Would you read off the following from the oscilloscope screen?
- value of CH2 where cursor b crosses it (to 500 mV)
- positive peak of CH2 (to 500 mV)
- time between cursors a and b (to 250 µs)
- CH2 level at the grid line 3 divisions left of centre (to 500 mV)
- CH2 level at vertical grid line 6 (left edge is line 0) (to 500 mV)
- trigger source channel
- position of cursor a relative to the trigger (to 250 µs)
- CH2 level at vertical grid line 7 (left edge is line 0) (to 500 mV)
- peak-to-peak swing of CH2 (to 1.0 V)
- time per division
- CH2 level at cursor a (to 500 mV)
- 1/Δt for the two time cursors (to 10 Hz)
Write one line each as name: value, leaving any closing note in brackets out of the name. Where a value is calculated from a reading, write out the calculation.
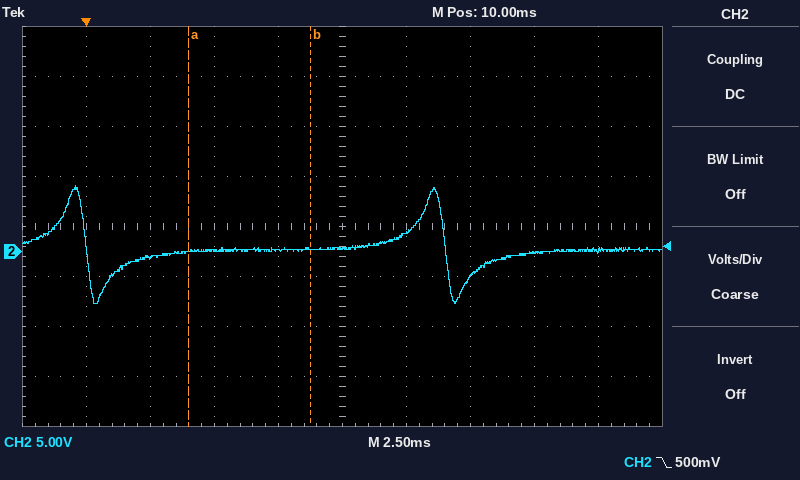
value of CH2 where cursor b crosses it: 500 mV
positive peak of CH2: 6.5 V
time between cursors a and b: 4.75 ms
CH2 level at the grid line 3 divisions left of centre: -500 mV
CH2 level at vertical grid line 6 (left edge is line 0): 2.0 V
trigger source channel: CH2
position of cursor a relative to the trigger: +4.00 ms
CH2 level at vertical grid line 7 (left edge is line 0): -2.5 V
peak-to-peak swing of CH2: 12.0 V
time per division: 2.5 ms
CH2 level at cursor a: 0.0 V
1/Δt for the two time cursors: 1 / 4.75 ms ≈ 210 Hz
